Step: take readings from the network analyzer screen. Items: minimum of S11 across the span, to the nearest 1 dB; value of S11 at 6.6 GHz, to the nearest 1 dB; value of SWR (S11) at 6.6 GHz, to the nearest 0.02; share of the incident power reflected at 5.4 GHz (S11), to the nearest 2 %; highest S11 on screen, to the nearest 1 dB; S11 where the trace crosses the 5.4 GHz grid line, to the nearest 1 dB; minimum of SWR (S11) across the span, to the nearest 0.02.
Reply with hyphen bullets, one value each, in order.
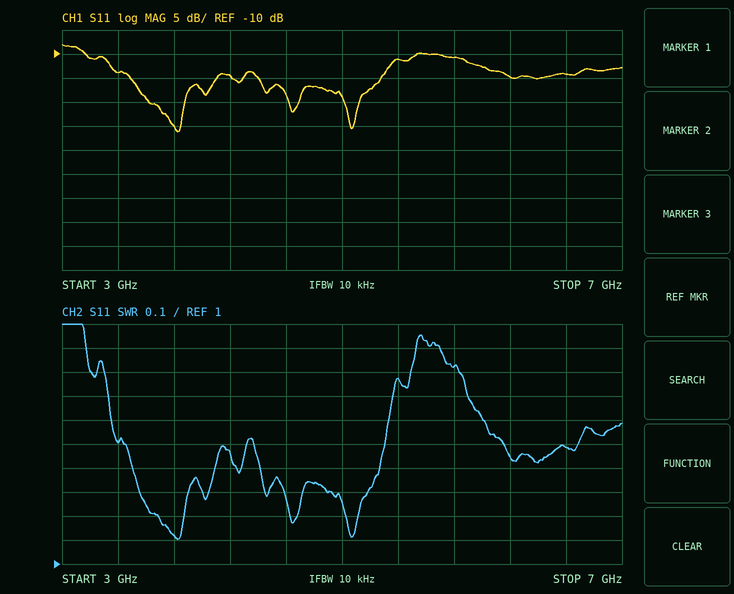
- -26 dB
- -14 dB
- 1.48
- 8 %
- -8 dB
- -11 dB
- 1.10
